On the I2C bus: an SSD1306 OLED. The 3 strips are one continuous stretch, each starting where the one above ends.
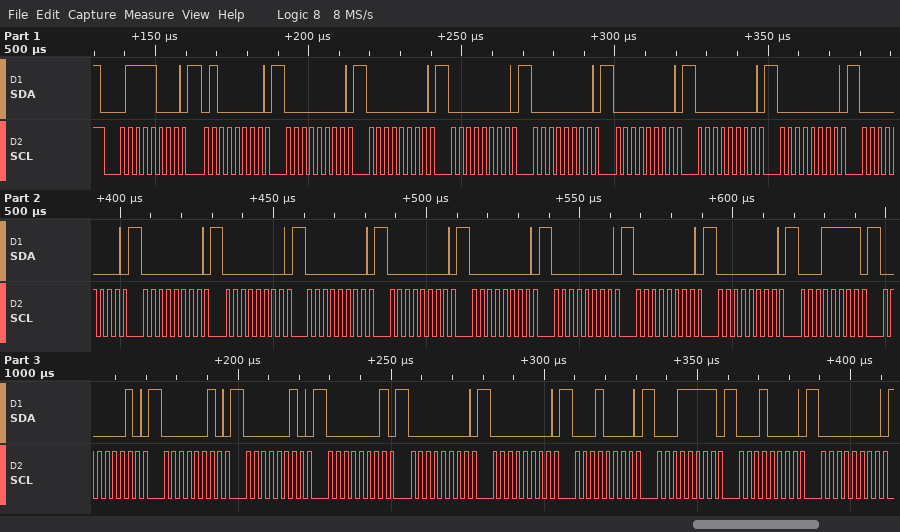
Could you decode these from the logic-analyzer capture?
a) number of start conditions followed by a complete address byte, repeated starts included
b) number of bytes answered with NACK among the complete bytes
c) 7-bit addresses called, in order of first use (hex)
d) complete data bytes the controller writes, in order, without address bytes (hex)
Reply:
1
0
0x3C
40 00 00 00 00 00 00 00 00 00 00 00 00 00 00 00 00 1F 02 02 02 01 00 00 10 1F 10 00
